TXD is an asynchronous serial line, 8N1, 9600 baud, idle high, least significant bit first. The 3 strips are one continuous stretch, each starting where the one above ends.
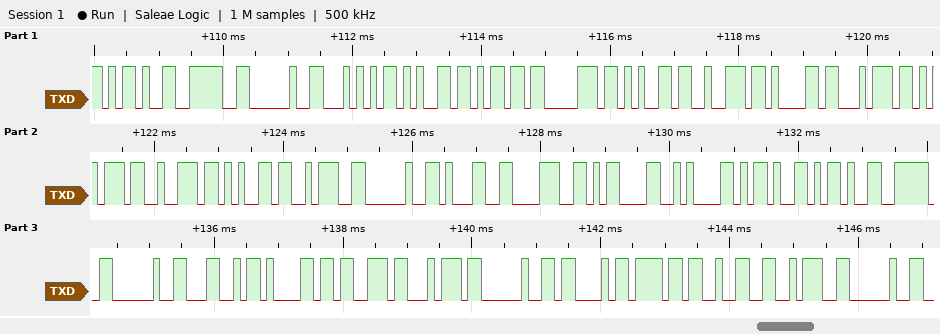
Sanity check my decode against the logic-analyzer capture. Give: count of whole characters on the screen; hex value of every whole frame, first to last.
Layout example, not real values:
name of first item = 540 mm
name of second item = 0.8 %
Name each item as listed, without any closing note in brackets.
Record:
count of whole characters on the screen = 34
hex value of every whole frame, first to last = 0x2D 0x3E 0x20 0x54 0x65 0x6D 0x70 0x65 0x72 0x61 0x74 0x75 0x72 0x65 0x3A 0x20 0x31 0x38 0x0D 0x0A 0x2D 0x2D 0x3E 0x20 0x4C 0x61 0x73 0x74 0x20 0x43 0x6F 0x32 0x3A 0x20
